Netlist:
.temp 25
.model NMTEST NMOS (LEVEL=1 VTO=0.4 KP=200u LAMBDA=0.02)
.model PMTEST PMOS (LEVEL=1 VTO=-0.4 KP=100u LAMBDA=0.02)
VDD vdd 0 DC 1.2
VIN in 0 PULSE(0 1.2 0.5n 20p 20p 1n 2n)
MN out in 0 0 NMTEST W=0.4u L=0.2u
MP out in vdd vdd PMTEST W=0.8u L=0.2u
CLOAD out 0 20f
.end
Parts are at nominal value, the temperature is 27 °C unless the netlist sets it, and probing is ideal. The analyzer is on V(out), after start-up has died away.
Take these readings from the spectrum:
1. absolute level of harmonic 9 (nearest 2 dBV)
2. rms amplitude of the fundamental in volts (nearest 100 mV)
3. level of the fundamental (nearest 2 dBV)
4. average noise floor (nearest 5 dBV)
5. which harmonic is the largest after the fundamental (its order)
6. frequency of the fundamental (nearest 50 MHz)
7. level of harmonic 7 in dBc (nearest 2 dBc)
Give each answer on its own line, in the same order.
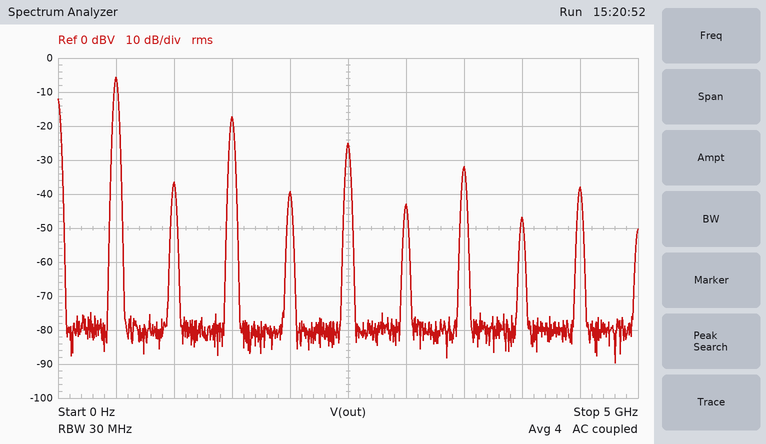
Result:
-38 dBV
500 mV
-6 dBV
-80 dBV
3
500 MHz
-26 dBc
